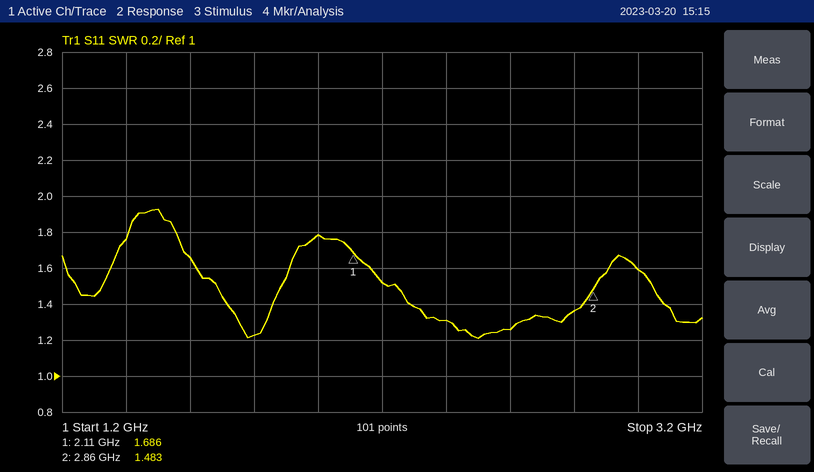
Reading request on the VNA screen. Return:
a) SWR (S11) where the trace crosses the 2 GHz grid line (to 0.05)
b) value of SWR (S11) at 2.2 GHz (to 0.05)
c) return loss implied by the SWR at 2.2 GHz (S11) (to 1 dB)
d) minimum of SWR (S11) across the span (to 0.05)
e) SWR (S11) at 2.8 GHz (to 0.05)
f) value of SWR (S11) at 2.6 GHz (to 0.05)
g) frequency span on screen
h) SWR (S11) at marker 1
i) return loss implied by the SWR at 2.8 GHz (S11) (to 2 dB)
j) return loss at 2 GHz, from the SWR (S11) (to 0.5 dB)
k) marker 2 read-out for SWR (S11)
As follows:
1.80
1.50
14 dB
1.20
1.35
1.25
2 GHz
1.686
16 dB
11.0 dB
1.483
